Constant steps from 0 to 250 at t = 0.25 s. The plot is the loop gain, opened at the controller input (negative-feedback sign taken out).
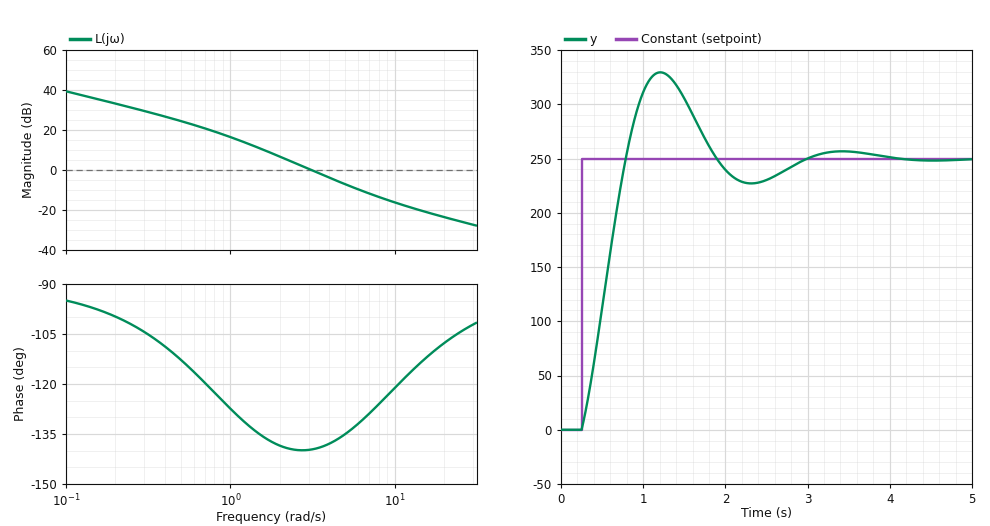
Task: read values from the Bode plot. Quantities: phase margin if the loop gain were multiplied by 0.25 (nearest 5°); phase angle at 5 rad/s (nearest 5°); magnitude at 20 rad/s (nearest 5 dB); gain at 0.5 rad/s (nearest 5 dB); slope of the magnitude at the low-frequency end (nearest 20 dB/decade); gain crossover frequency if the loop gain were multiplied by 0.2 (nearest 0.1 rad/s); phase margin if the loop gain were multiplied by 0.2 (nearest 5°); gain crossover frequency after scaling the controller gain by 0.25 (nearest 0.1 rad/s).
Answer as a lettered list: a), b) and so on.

a) 45°
b) -135°
c) -25 dB
d) 25 dB
e) -20 dB/decade
f) 1.2 rad/s
g) 50°
h) 1.4 rad/s
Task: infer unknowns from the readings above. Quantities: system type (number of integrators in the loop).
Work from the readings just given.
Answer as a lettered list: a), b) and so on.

a) 1
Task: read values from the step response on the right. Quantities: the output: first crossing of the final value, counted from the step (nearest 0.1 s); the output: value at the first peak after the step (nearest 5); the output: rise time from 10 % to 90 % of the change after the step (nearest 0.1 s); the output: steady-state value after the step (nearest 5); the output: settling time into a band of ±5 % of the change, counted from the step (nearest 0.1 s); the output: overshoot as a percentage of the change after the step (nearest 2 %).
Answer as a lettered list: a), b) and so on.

a) 0.5 s
b) 330
c) 0.4 s
d) 250
e) 2.4 s
f) 32 %
